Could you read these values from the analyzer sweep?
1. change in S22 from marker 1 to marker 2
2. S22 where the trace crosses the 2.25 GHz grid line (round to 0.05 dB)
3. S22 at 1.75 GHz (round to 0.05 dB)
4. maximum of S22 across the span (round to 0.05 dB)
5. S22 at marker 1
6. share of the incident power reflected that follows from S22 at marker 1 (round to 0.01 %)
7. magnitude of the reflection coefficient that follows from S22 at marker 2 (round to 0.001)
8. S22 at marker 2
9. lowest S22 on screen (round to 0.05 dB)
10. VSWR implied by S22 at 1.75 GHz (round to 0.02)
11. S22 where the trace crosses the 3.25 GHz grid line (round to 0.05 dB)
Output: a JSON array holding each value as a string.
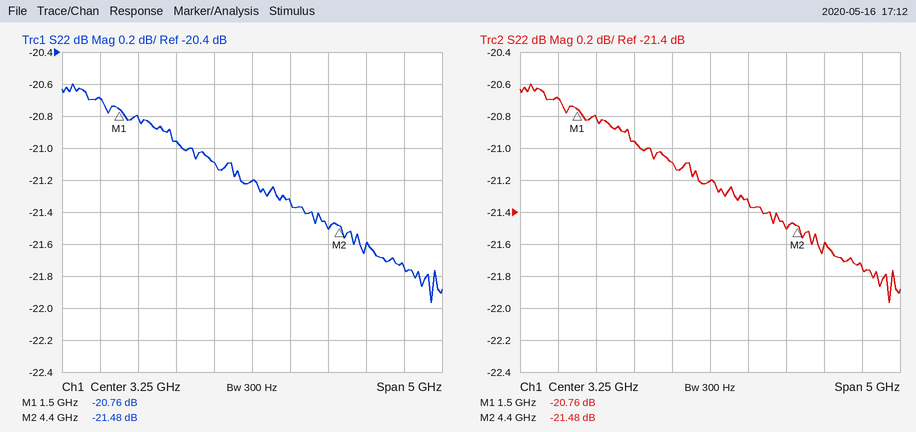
["-0.72 dB", "-20.95 dB", "-20.80 dB", "-20.60 dB", "-20.76 dB", "0.84 %", "0.084", "-21.48 dB", "-21.95 dB", "1.20", "-21.20 dB"]
